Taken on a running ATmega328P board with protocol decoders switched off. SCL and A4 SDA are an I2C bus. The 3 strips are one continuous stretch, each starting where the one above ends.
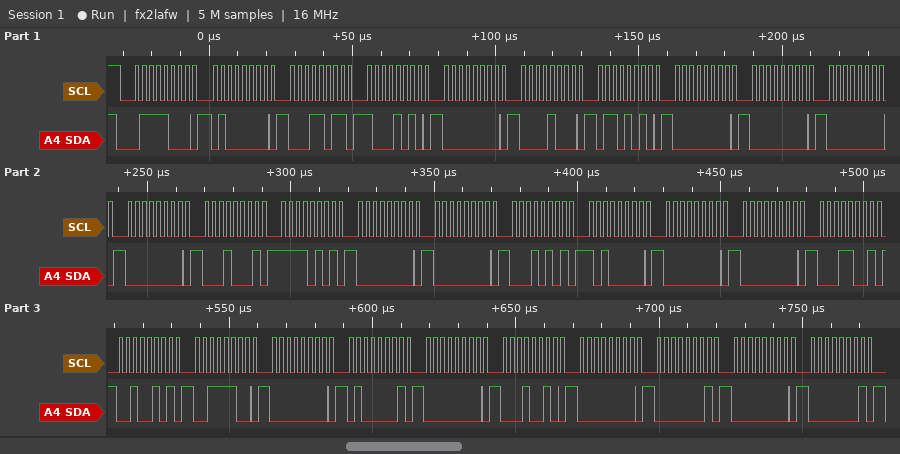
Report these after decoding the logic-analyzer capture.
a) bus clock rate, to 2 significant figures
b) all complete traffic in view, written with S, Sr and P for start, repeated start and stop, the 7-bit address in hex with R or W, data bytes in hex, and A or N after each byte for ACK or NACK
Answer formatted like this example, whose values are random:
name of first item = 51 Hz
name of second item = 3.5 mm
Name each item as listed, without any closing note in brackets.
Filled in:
bus clock rate, to 2 significant figures = 400 kHz
all complete traffic in view, written with S, Sr and P for start, repeated start and stop, the 7-bit address in hex with R or W, data bytes in hex, and A or N after each byte for ACK or NACK = S 3CW A 40 A 1B A 8A A 00 A 08 A 6A A 00 A 00 A 00 A 00 A 11 A F5 A 00 A 00 A 15 A A0 A 00 A 00 A 19 A 25 A 3C A 00 A 41 A 00 A 12 A 00 A 01 A 00 A 01 A
